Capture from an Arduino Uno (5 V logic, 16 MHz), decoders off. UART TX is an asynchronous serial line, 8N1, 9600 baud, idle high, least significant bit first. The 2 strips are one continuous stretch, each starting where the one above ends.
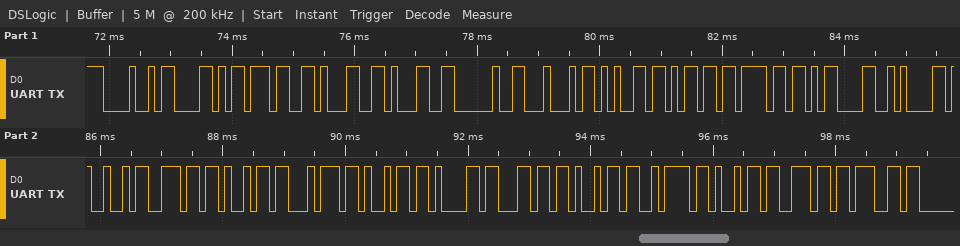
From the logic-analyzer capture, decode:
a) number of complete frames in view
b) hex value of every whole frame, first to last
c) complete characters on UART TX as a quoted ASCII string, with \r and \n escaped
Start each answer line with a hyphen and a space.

- 24
- 48 58 37 31 31 20 44 65 6D 6F 0D 0A 49 6E 69 74 69 61 6C 69 7A 69 6E 67
- "HX711 Demo\r\nInitializing"
